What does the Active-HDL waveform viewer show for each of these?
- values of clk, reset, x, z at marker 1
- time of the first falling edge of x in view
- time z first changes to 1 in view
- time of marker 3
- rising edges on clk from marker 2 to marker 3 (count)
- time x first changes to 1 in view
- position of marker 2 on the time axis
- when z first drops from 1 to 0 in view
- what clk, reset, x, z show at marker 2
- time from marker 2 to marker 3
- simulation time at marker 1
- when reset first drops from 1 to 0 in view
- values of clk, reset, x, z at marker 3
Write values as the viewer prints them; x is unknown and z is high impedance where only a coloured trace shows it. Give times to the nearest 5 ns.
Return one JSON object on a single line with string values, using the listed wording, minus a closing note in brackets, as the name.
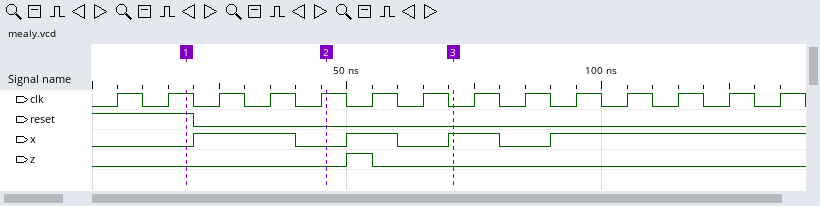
{"values of clk, reset, x, z at marker 1": "clk=1, reset=1, x=0, z=0", "time of the first falling edge of x in view": "40 ns", "time z first changes to 1 in view": "50 ns", "time of marker 3": "70 ns", "rising edges on clk from marker 2 to marker 3": "2", "time x first changes to 1 in view": "20 ns", "position of marker 2 on the time axis": "45 ns", "when z first drops from 1 to 0 in view": "55 ns", "what clk, reset, x, z show at marker 2": "clk=1, reset=0, x=0, z=0", "time from marker 2 to marker 3": "25 ns", "simulation time at marker 1": "20 ns", "when reset first drops from 1 to 0 in view": "20 ns", "values of clk, reset, x, z at marker 3": "clk=0, reset=0, x=1, z=0"}
